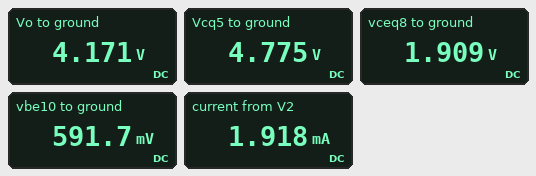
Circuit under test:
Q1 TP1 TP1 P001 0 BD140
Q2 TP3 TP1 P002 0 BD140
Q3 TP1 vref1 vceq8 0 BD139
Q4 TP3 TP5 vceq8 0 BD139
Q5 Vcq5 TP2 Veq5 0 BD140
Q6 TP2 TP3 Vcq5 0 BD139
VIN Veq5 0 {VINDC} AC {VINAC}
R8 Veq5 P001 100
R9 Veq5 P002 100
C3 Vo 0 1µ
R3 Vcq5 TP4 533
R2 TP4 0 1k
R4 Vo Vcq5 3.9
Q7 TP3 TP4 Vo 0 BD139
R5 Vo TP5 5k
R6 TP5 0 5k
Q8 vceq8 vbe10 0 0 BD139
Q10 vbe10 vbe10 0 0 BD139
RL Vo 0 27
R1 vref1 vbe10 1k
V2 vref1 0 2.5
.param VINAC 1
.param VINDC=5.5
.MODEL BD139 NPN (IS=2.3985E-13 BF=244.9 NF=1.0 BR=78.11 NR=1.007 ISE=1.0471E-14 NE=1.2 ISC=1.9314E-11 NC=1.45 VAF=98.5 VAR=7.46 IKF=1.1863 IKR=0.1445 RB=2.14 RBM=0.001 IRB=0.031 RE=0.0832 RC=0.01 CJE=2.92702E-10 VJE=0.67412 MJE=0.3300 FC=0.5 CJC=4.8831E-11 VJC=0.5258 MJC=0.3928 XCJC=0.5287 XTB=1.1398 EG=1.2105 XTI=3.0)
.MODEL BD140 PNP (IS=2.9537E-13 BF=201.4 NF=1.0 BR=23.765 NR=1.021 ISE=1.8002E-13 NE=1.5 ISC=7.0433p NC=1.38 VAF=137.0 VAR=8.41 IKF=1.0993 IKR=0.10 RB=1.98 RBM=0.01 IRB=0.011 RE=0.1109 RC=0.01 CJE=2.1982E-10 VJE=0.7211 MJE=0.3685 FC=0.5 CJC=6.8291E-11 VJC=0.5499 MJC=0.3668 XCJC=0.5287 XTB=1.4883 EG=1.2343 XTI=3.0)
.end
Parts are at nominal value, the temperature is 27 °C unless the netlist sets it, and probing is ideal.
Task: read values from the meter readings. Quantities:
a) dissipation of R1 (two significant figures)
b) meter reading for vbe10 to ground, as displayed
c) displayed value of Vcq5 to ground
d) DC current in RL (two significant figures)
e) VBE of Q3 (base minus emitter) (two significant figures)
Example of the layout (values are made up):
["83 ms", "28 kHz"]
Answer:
["3.6 mW", "591.7 mV", "4.775 V", "150 mA", "590 mV"]
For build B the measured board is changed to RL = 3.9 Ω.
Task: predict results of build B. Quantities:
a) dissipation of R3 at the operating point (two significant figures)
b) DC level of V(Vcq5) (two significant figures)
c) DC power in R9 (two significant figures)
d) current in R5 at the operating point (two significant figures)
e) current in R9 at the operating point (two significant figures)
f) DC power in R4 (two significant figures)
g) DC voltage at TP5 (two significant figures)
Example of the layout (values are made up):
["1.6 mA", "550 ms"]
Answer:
["3.5 mW", "3.9 V", "360 µW", "200 µA", "1.9 mA", "980 mW", "980 mV"]
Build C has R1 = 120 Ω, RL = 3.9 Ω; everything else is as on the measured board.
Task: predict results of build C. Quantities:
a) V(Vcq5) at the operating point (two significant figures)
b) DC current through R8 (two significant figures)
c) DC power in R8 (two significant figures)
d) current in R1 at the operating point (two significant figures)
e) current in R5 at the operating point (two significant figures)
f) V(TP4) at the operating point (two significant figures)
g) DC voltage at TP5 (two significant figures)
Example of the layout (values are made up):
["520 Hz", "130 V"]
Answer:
["4.0 V", "9.4 mA", "8.9 mW", "15 mA", "200 µA", "2.6 V", "1.0 V"]
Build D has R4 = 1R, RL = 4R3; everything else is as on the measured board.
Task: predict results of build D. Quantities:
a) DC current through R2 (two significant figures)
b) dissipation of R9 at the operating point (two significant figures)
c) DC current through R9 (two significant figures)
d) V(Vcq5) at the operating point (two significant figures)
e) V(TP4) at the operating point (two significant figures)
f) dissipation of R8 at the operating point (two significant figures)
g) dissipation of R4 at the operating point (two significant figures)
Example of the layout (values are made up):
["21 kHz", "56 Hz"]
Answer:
["3.0 mA", "300 µW", "1.7 mA", "4.6 V", "3.0 V", "330 µW", "760 mW"]
